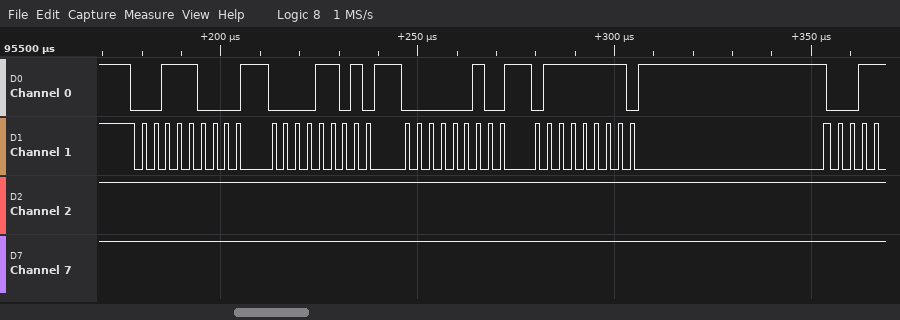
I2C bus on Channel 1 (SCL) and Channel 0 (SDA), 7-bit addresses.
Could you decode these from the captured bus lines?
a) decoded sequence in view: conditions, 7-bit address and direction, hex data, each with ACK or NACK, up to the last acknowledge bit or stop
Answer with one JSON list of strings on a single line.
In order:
["start, address 1C write ACK, 0D ACK, 02 ACK, 7F ACK"]
